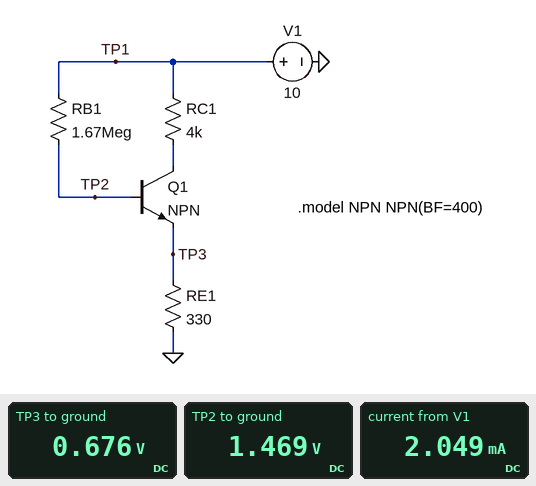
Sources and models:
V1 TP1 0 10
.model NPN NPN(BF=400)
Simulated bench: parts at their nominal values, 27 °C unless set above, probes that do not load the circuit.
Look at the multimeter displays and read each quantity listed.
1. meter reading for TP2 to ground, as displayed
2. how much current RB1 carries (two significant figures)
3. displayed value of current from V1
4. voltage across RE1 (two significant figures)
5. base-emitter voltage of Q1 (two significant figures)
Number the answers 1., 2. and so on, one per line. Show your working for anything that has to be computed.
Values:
1. 1.469 V
2. (10 V - 1.469 V) / 1.67 MΩ = 5.1 µA
3. 2.049 mA
4. 676 mV = 680 mV
5. 1.469 V - 676 mV = 790 mV
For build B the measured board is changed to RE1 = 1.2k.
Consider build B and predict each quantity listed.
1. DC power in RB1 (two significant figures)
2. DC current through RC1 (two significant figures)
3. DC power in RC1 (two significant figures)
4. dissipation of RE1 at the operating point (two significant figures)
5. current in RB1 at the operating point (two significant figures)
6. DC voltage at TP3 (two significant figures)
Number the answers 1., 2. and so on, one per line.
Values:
1. 31 µW
2. 1.7 mA
3. 12 mW
4. 3.5 mW
5. 4.3 µA
6. 2.1 V
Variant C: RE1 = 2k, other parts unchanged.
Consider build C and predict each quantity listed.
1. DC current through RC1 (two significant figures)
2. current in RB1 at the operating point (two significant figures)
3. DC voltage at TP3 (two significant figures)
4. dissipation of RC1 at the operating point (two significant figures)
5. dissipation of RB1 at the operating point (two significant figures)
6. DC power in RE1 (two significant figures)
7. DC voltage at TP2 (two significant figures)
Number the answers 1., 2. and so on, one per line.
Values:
1. 1.5 mA
2. 3.7 µA
3. 3.0 V
4. 8.9 mW
5. 23 µW
6. 4.5 mW
7. 3.8 V
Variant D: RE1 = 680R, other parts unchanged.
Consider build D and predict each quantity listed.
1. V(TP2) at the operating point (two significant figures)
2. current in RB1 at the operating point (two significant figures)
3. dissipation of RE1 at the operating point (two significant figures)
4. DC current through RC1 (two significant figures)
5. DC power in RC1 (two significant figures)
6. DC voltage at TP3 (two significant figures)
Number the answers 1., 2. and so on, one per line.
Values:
1. 2.1 V
2. 4.7 µA
3. 2.5 mW
4. 1.9 mA
5. 14 mW
6. 1.3 V
